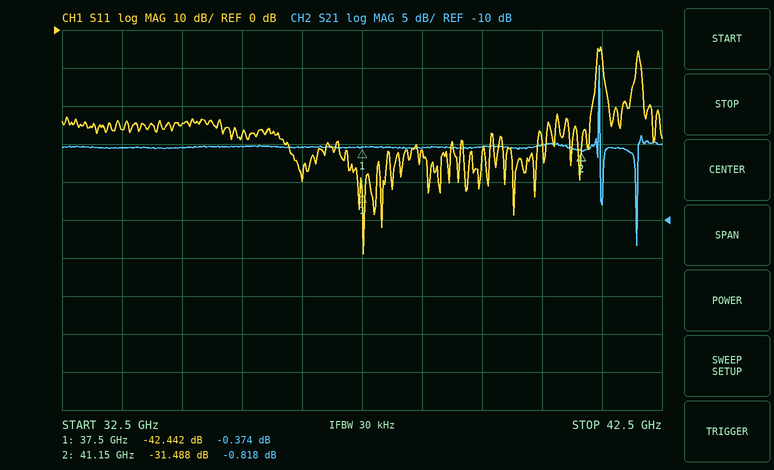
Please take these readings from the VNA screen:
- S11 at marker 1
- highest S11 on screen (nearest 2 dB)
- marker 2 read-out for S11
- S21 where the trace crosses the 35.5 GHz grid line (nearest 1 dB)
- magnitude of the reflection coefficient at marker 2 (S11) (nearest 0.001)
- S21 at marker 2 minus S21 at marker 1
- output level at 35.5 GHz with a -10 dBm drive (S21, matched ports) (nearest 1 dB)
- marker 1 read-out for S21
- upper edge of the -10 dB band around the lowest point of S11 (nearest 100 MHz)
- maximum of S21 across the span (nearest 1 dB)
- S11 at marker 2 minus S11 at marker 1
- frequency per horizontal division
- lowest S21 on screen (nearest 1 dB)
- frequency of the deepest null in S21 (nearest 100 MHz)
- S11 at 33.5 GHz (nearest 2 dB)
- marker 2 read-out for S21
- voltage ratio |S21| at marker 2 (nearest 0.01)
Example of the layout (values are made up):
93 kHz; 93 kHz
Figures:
-42.442 dB; -4 dB; -31.488 dB; 0 dB; 0.027; -0.444 dB; -10 dBm; -0.374 dB; 41.4 GHz; 10 dB; 10.954 dB; 1 GHz; -13 dB; 42.1 GHz; -26 dB; -0.818 dB; 0.91
